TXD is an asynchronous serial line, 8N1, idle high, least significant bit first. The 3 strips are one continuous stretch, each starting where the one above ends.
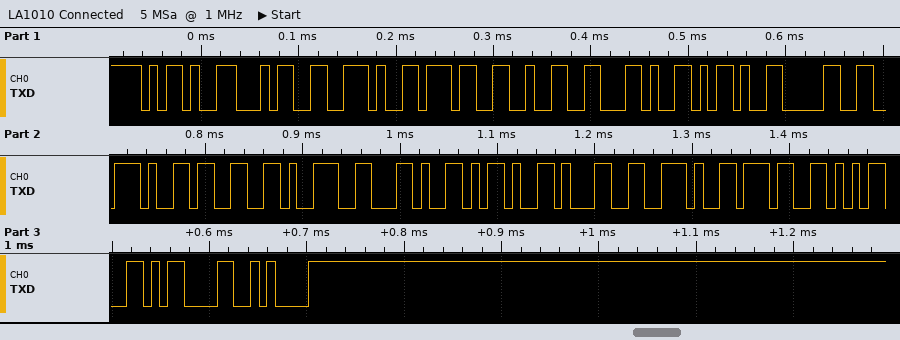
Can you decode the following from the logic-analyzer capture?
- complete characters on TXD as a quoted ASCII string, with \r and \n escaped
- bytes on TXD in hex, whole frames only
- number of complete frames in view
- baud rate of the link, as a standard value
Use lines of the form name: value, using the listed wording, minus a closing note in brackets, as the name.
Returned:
complete characters on TXD as a quoted ASCII string, with \r and \n escaped: "-4.72,-0.39,-1.75\r\n"
bytes on TXD in hex, whole frames only: 0x2D 0x34 0x2E 0x37 0x32 0x2C 0x2D 0x30 0x2E 0x33 0x39 0x2C 0x2D 0x31 0x2E 0x37 0x35 0x0D 0x0A
number of complete frames in view: 19
baud rate of the link, as a standard value: 115200 baud
